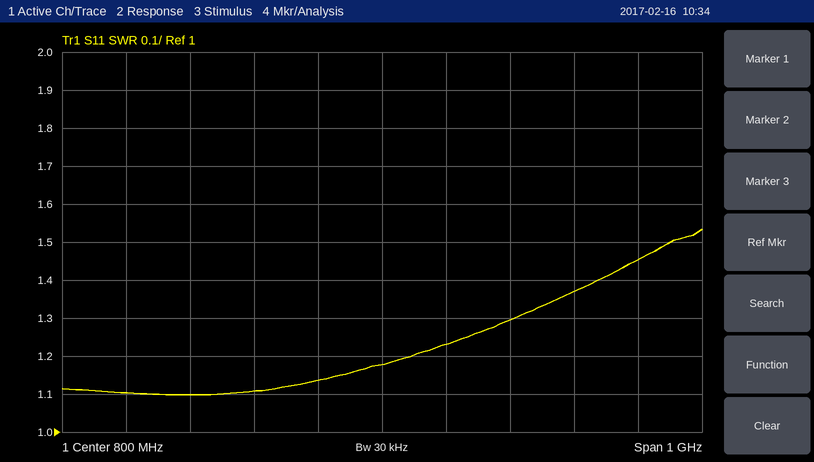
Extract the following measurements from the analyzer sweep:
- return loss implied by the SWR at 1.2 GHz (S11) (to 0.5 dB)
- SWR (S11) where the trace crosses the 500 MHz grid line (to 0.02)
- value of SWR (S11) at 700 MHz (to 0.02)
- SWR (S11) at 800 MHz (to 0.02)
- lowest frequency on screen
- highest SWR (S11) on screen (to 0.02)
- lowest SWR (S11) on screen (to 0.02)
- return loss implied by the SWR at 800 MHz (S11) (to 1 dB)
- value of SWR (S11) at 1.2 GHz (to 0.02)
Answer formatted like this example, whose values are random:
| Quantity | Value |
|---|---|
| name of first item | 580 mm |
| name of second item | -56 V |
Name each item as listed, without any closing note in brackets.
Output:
| Quantity | Value |
|---|---|
| return loss implied by the SWR at 1.2 GHz (S11) | 14.5 dB |
| SWR (S11) where the trace crosses the 500 MHz grid line | 1.10 |
| value of SWR (S11) at 700 MHz | 1.14 |
| SWR (S11) at 800 MHz | 1.18 |
| lowest frequency on screen | 300 MHz |
| highest SWR (S11) on screen | 1.54 |
| lowest SWR (S11) on screen | 1.10 |
| return loss implied by the SWR at 800 MHz (S11) | 22 dB |
| value of SWR (S11) at 1.2 GHz | 1.46 |
